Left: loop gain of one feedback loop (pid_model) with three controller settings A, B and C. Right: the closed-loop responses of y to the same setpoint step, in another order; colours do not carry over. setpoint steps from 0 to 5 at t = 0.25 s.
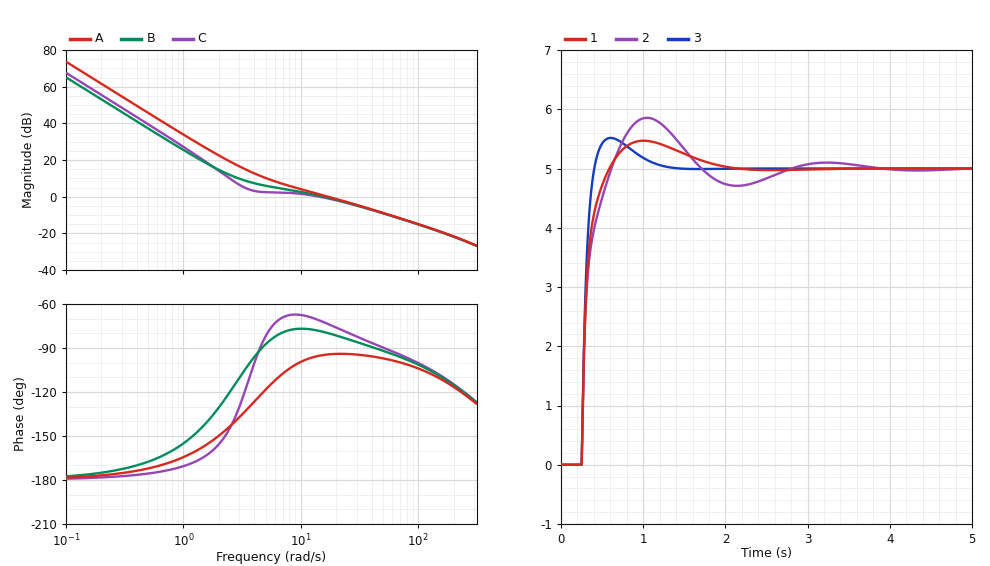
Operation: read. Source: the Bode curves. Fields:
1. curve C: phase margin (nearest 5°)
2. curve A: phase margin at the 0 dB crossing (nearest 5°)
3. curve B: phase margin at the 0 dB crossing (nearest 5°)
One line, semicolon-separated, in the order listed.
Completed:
110°; 85°; 100°
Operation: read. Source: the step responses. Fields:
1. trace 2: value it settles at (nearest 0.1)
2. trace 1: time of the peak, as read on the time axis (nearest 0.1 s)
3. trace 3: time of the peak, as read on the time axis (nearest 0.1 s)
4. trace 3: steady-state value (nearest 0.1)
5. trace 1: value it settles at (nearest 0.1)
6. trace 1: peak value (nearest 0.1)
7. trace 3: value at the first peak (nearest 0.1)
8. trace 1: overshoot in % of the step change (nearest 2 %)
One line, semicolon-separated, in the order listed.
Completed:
5.0; 1.0 s; 0.6 s; 5.0; 5.0; 5.5; 5.5; 10 %
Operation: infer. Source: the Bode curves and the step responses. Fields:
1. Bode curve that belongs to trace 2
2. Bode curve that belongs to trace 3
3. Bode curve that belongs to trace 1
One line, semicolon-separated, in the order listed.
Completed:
C; A; B
